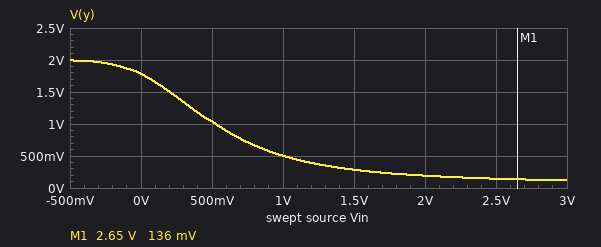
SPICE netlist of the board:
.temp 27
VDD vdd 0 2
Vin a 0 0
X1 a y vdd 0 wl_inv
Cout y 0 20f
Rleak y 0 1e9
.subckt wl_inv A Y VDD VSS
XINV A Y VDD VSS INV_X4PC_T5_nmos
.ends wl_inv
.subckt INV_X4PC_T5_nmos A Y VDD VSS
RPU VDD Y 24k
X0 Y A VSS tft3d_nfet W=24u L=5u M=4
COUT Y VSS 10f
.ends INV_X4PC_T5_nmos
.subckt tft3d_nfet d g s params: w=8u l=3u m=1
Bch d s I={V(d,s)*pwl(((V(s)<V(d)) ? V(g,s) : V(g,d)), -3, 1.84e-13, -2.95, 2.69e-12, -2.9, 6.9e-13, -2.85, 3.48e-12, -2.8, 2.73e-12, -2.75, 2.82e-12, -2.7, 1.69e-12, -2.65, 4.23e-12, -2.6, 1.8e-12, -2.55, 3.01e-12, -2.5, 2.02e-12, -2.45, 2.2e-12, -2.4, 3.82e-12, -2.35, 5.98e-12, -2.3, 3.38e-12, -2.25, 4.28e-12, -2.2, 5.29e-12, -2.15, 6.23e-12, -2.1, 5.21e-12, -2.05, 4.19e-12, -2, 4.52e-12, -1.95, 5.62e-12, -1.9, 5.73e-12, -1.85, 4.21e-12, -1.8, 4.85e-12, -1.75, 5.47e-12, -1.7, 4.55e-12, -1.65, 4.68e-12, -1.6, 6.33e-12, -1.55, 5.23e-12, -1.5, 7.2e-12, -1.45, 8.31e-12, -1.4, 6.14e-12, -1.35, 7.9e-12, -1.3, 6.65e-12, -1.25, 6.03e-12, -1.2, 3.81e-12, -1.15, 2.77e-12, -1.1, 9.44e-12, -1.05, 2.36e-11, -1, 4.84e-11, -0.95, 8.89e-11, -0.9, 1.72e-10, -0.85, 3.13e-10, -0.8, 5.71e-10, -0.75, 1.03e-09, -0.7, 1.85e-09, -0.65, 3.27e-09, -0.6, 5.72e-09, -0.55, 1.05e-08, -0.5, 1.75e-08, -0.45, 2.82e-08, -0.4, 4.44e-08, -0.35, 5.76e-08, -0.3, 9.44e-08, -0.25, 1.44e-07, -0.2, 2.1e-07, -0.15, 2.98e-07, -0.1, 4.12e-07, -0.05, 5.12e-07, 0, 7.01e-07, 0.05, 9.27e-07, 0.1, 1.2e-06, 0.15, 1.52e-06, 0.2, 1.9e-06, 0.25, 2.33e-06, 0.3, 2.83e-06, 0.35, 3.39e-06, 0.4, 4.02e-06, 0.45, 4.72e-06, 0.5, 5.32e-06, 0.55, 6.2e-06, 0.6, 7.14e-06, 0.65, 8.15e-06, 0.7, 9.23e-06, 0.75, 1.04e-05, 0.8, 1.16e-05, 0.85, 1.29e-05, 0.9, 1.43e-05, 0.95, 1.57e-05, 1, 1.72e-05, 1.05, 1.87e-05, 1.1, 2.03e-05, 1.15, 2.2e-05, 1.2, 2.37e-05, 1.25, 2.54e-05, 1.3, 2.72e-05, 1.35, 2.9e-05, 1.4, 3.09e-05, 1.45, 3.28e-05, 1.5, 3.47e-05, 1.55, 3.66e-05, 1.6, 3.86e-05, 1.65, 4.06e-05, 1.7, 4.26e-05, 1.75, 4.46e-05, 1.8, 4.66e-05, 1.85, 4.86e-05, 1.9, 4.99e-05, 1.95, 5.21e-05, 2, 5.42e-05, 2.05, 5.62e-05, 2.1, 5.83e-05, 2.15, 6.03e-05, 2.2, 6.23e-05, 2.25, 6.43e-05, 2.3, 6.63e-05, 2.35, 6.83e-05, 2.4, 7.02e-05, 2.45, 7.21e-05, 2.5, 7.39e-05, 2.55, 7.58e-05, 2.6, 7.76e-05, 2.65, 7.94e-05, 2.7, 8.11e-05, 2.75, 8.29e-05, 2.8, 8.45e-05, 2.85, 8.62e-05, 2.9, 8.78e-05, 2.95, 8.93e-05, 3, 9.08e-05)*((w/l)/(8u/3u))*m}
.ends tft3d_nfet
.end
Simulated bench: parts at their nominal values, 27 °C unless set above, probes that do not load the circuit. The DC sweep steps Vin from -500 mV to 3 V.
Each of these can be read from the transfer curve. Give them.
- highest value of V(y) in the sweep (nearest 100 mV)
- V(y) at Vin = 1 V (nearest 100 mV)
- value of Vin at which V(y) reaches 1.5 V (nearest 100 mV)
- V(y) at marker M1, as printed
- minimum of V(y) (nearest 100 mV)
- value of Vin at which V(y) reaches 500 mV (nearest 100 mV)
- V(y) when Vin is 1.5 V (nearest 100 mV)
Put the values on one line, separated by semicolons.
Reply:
2.0 V; 500 mV; 200 mV; 136 mV; 100 mV; 1.0 V; 300 mV
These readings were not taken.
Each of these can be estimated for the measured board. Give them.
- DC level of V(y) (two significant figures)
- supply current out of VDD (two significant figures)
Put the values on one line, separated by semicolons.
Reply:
1.8 V; 9.0 µA
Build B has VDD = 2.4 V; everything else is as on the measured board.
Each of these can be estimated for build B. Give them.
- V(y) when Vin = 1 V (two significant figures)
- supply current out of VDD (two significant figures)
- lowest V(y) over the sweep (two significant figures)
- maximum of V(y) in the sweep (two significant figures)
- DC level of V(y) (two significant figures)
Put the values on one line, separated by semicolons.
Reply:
600 mV; 11 µA; 140 mV; 2.4 V; 2.1 V
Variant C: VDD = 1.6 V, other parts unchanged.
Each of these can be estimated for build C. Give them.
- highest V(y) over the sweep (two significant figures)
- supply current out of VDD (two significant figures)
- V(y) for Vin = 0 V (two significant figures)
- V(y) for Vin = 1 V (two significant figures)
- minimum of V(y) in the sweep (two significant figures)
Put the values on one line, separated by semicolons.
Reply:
1.6 V; 7.2 µA; 1.4 V; 400 mV; 96 mV
